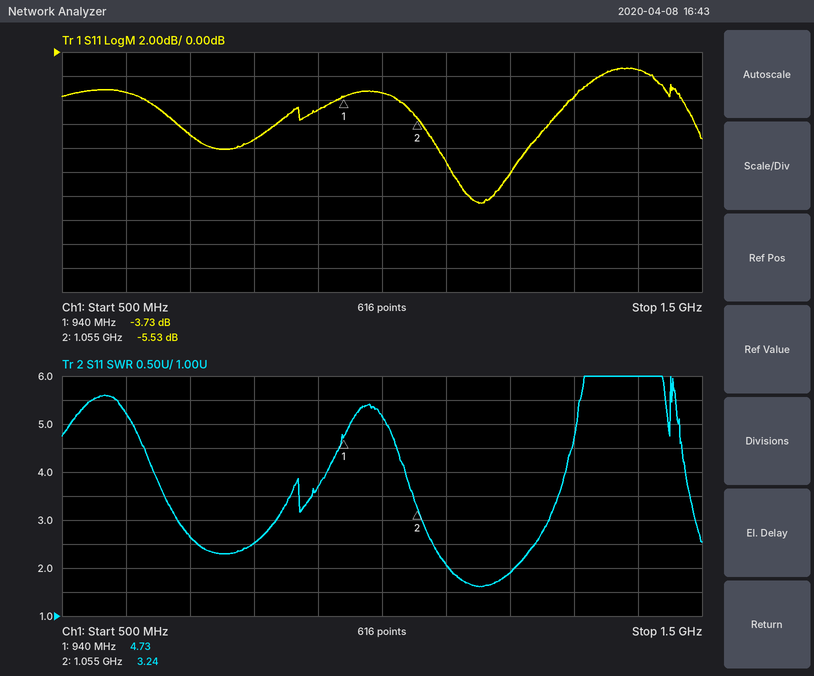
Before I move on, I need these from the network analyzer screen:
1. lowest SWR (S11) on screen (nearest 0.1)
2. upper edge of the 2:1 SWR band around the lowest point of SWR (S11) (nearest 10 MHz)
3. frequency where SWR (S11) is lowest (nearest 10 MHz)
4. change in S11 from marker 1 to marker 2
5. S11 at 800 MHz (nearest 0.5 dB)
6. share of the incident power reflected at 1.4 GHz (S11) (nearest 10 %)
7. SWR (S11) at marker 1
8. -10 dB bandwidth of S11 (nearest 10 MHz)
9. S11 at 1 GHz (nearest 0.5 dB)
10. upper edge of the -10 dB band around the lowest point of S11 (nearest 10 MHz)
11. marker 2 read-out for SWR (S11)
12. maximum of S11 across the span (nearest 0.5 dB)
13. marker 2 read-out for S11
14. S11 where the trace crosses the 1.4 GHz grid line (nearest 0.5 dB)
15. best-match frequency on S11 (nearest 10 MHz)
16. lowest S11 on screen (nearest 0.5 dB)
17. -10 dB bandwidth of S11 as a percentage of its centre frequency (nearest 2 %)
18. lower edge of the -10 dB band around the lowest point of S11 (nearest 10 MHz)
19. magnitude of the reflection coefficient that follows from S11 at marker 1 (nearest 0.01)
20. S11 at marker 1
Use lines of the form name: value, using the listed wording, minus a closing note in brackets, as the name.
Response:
lowest SWR (S11) on screen: 1.6
upper edge of the 2:1 SWR band around the lowest point of SWR (S11): 1.21 GHz
frequency where SWR (S11) is lowest: 1.15 GHz
change in S11 from marker 1 to marker 2: -1.80 dB
S11 at 800 MHz: -7.5 dB
share of the incident power reflected at 1.4 GHz (S11): 70 %
SWR (S11) at marker 1: 4.73
-10 dB bandwidth of S11: 90 MHz
S11 at 1 GHz: -3.5 dB
upper edge of the -10 dB band around the lowest point of S11: 1.20 GHz
marker 2 read-out for SWR: 3.24
maximum of S11 across the span: -1.5 dB
marker 2 read-out for S11: -5.53 dB
S11 where the trace crosses the 1.4 GHz grid line: -1.5 dB
best-match frequency on S11: 1.15 GHz
lowest S11 on screen: -12.5 dB
-10 dB bandwidth of S11 as a percentage of its centre frequency: 8 %
lower edge of the -10 dB band around the lowest point of S11: 1.11 GHz
magnitude of the reflection coefficient that follows from S11 at marker 1: 0.65
S11 at marker 1: -3.73 dB
